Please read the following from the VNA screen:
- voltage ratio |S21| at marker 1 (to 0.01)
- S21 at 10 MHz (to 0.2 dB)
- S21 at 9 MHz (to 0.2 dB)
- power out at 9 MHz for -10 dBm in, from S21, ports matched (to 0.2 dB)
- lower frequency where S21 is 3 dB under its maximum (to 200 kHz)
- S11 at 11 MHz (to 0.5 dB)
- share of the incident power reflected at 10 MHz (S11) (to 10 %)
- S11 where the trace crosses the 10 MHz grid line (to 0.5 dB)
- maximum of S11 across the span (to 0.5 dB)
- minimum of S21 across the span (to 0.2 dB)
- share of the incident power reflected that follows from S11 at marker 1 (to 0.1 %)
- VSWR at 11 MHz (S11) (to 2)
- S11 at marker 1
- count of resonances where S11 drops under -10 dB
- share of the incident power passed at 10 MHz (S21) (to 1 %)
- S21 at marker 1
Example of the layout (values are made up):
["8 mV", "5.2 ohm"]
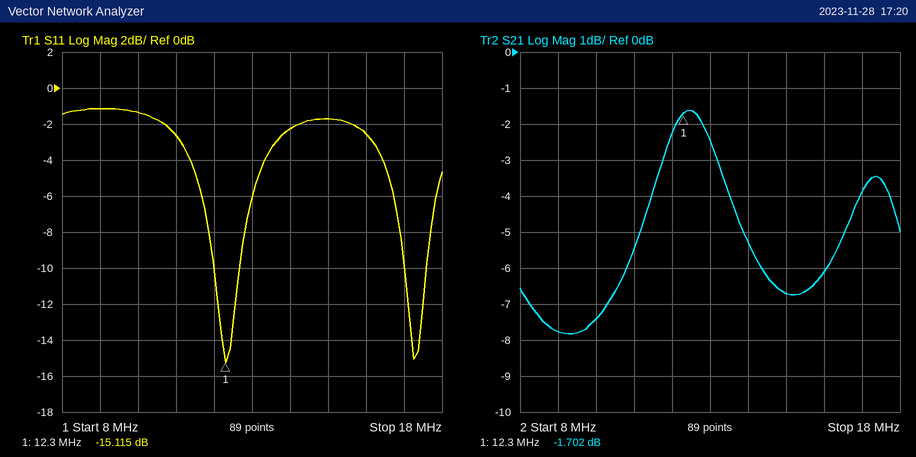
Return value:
["0.82", "-7.4 dB", "-7.8 dB", "-17.8 dBm", "11.2 MHz", "-2.5 dB", "70 %", "-1.5 dB", "-1.0 dB", "-7.8 dB", "3.1 %", "6", "-15.115 dB", "2", "18 %", "-1.702 dB"]
